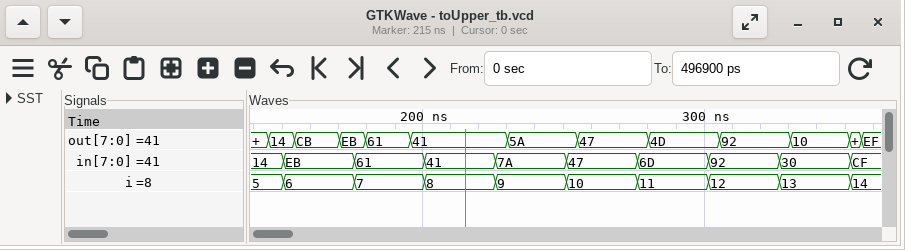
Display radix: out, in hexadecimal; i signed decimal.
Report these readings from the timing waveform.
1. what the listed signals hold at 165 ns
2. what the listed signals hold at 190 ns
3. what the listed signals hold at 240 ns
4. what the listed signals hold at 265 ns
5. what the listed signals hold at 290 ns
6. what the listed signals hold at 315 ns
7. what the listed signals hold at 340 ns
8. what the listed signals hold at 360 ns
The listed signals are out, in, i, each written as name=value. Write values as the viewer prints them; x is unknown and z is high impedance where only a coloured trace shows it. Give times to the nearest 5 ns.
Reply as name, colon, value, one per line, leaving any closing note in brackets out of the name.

what the listed signals hold at 165 ns: out=CB, in=EB, i=6
what the listed signals hold at 190 ns: out=61, in=61, i=7
what the listed signals hold at 240 ns: out=5A, in=7A, i=9
what the listed signals hold at 265 ns: out=47, in=47, i=10
what the listed signals hold at 290 ns: out=4D, in=6D, i=11
what the listed signals hold at 315 ns: out=92, in=92, i=12
what the listed signals hold at 340 ns: out=10, in=30, i=13
what the listed signals hold at 360 ns: out=EF, in=CF, i=14
